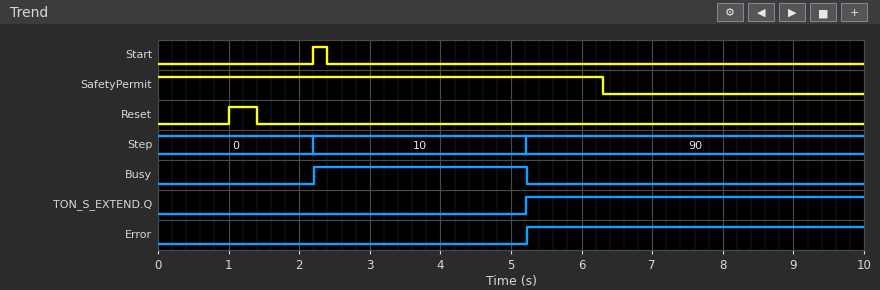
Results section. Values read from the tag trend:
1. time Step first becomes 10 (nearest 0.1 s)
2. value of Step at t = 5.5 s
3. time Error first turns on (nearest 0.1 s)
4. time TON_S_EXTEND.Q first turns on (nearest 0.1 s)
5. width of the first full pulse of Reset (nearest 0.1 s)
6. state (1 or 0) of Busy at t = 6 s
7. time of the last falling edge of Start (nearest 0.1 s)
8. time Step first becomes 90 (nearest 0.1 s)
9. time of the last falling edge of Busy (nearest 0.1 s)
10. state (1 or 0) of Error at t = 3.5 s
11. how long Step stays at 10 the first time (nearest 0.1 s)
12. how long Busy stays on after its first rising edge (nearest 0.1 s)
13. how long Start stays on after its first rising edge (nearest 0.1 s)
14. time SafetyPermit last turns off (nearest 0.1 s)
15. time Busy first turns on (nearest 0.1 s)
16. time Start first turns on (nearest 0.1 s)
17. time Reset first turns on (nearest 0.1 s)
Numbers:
2.2 s
90
5.2 s
5.2 s
0.4 s
0
2.4 s
5.2 s
5.2 s
0
3.0 s
3.0 s
0.2 s
6.3 s
2.2 s
2.2 s
1.0 s
